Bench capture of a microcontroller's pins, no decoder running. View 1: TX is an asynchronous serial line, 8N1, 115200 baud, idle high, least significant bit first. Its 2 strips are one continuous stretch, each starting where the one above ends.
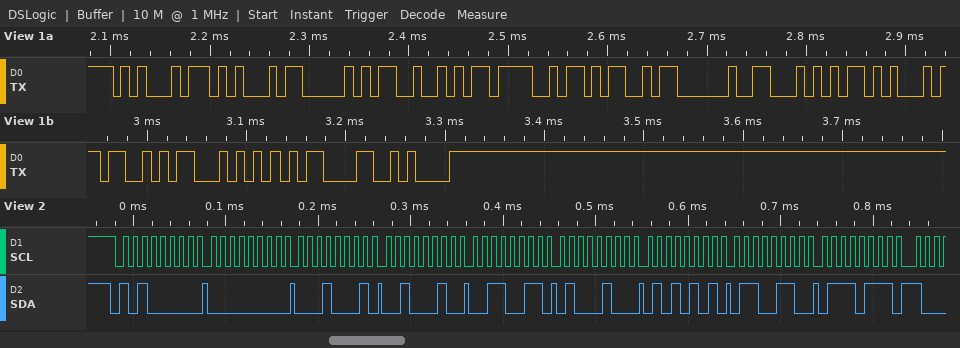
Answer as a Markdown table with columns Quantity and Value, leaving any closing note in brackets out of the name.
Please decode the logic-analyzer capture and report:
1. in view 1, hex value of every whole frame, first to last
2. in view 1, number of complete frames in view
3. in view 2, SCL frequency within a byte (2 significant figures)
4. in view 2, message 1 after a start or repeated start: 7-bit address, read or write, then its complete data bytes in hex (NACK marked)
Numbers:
| Quantity | Value |
|---|---|
| in view 1, hex value of every whole frame, first to last | 0x45 0x45 0x50 0x52 0x4F 0x4D 0x20 0x54 0x45 0x53 0x54 0x0D 0x0A |
| in view 1, number of complete frames in view | 13 |
| in view 2, SCL frequency within a byte | 100 kHz |
| in view 2, message 1 after a start or repeated start: 7-bit address, read or write, then its complete data bytes in hex | 0x50 write: 00 11 22 33 44 55 66 77 |
